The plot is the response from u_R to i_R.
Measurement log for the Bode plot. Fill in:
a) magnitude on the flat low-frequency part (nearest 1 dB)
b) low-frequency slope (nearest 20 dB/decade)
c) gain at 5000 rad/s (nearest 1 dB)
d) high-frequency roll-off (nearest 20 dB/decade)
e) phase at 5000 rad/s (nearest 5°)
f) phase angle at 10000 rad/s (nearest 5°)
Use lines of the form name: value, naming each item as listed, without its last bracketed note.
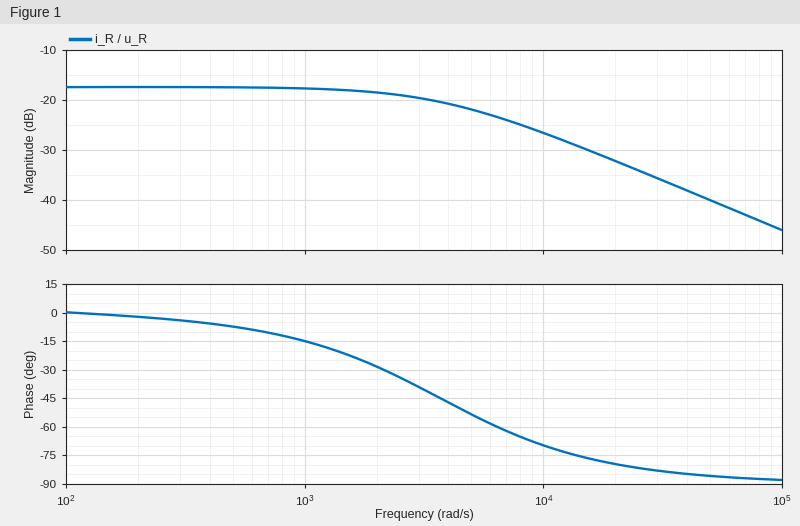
magnitude on the flat low-frequency part: -17 dB
low-frequency slope: 0 dB/decade
gain at 5000 rad/s: -22 dB
high-frequency roll-off: -20 dB/decade
phase at 5000 rad/s: -55°
phase angle at 10000 rad/s: -70°
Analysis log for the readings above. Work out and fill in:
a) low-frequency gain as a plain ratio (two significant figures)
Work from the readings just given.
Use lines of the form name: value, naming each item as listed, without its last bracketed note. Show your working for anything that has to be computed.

low-frequency gain as a plain ratio: 10^(-17 / 20) = 0.14
